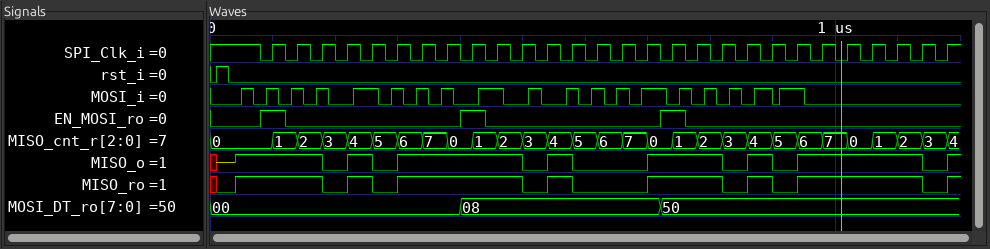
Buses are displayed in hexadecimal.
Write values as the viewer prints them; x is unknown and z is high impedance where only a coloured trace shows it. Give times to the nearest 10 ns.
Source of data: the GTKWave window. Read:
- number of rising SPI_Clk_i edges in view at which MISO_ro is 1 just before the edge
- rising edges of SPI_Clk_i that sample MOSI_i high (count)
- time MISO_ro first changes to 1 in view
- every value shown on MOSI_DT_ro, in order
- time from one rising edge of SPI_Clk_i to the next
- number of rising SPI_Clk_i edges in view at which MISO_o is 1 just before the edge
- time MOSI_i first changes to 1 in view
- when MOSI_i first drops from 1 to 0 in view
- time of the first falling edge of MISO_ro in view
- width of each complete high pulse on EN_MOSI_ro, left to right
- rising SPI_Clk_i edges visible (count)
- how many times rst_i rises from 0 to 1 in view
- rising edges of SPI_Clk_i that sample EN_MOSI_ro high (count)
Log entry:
19
14
40 ns
00, 08, 50
40 ns
19
50 ns
70 ns
180 ns
40 ns, 40 ns, 40 ns
28
1
3
